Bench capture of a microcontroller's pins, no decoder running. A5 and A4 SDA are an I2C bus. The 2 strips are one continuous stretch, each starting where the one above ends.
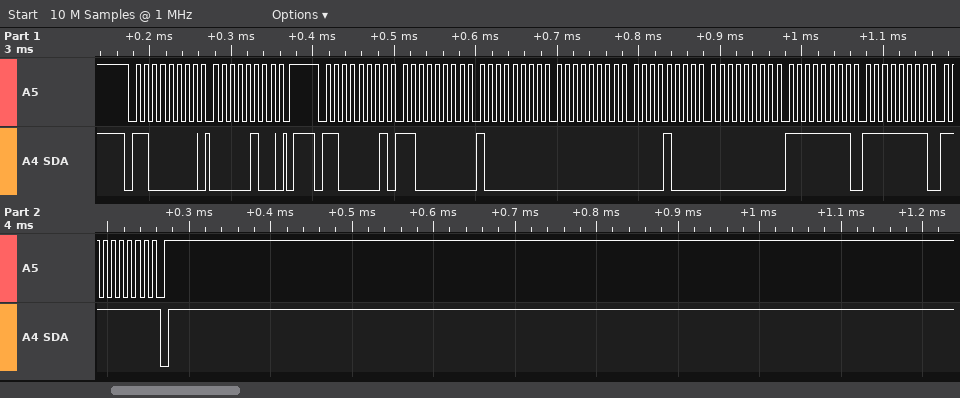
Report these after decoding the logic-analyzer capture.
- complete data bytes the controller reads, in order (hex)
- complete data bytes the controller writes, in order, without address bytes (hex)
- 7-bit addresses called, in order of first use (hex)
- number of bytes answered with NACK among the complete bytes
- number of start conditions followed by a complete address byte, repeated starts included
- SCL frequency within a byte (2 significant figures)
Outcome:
C0 80 00 08 00 FF FF FF
04
0x60
1
2
100 kHz
